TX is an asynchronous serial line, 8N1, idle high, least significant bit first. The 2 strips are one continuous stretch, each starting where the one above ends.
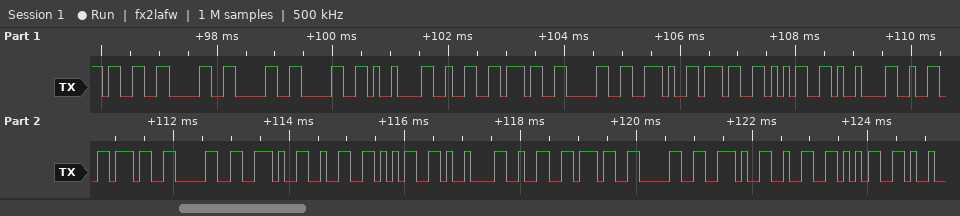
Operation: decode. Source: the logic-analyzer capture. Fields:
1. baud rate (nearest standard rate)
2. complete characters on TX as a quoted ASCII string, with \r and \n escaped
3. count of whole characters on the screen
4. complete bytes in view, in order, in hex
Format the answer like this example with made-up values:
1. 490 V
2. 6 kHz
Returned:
1. 9600 baud
2. "3000\t270.75\t270.25\t270.25"
3. 25
4. 0x33 0x30 0x30 0x30 0x09 0x32 0x37 0x30 0x2E 0x37 0x35 0x09 0x32 0x37 0x30 0x2E 0x32 0x35 0x09 0x32 0x37 0x30 0x2E 0x32 0x35
